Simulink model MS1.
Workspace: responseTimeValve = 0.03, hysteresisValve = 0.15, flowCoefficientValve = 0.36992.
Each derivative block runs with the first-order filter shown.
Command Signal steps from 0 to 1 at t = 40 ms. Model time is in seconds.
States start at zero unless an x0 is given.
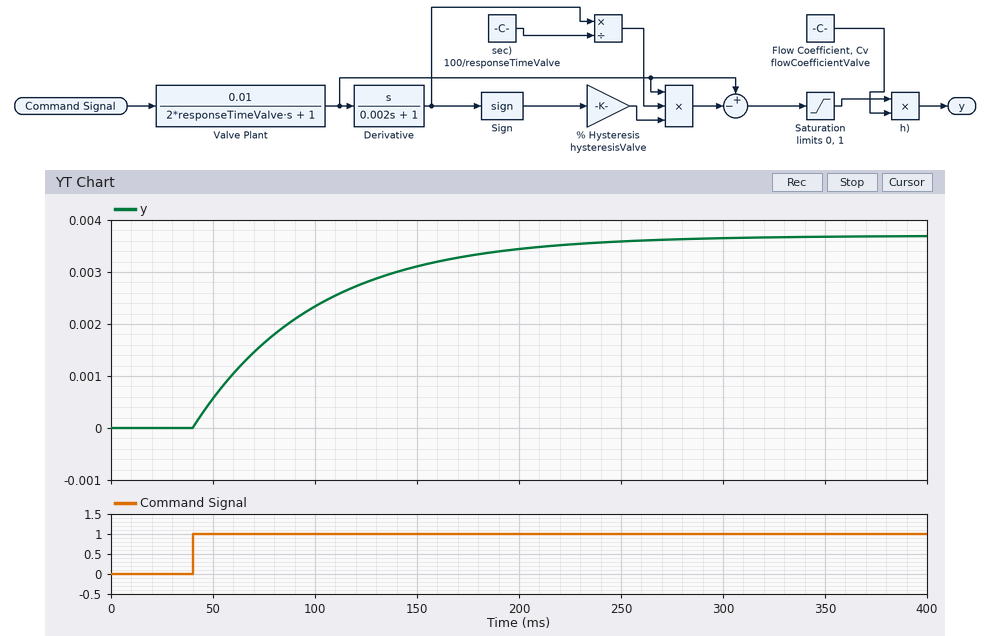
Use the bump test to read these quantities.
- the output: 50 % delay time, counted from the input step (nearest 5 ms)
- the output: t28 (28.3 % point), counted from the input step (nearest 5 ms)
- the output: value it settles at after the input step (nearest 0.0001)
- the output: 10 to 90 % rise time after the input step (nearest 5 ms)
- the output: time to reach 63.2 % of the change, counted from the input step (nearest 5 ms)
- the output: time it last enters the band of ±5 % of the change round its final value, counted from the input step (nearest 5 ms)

40 ms
20 ms
0.0037
130 ms
60 ms
180 ms
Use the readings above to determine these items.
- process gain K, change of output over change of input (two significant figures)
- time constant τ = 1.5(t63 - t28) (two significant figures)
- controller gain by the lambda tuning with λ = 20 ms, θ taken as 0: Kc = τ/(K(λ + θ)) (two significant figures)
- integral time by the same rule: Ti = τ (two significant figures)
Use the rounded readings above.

0.0037
60 ms
810
60 ms
